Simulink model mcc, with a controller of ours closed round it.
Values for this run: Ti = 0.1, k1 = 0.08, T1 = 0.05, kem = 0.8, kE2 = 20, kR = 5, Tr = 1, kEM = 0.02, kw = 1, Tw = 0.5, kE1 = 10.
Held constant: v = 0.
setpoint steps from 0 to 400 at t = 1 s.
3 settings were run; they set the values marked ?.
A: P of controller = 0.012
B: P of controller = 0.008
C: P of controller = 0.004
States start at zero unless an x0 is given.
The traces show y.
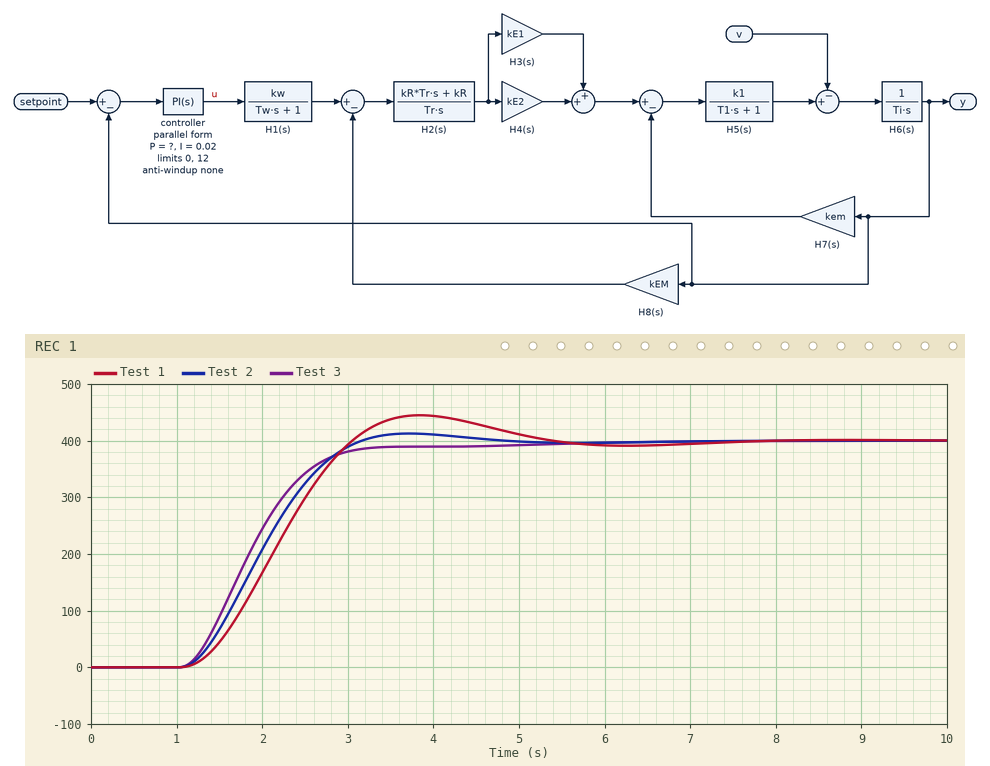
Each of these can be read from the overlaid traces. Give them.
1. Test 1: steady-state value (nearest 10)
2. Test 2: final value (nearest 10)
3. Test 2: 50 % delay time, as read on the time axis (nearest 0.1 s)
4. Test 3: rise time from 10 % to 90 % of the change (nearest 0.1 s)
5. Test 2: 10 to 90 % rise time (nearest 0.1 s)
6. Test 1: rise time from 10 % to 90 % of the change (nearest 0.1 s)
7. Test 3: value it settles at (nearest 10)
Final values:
400
400
2.0 s
1.3 s
1.3 s
1.3 s
400
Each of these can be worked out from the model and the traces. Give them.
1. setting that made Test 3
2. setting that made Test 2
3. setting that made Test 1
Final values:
A
B
C
